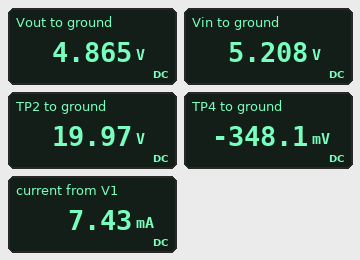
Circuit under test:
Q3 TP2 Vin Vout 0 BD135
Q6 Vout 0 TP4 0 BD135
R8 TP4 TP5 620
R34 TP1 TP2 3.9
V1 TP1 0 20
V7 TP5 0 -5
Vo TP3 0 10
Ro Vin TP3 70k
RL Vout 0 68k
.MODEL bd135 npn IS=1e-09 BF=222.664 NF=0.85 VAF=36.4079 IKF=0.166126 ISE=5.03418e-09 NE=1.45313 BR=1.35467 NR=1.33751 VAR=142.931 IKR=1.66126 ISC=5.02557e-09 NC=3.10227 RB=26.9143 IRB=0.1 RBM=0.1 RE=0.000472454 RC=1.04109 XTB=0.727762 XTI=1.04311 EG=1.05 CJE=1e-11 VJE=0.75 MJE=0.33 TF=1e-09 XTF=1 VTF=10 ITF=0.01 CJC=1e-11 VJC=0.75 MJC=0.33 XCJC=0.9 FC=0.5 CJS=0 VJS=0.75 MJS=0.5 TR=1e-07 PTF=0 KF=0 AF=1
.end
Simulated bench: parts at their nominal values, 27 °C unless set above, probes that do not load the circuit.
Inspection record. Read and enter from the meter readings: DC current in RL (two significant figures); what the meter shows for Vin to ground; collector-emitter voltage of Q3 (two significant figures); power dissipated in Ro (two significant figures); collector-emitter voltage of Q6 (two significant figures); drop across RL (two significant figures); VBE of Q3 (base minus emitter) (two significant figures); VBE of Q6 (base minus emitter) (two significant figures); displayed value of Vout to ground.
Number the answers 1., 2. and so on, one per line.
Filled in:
1. 72 µA
2. 5.208 V
3. 15 V
4. 330 µW
5. 5.2 V
6. 4.9 V
7. 340 mV
8. 350 mV
9. 4.865 V
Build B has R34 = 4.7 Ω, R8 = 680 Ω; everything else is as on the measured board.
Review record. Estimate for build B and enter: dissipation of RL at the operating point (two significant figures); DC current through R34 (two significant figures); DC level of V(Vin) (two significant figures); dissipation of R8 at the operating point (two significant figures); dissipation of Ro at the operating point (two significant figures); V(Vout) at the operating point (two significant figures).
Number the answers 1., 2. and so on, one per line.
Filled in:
1. 390 µW
2. 6.8 mA
3. 5.5 V
4. 32 mW
5. 290 µW
6. 5.2 V
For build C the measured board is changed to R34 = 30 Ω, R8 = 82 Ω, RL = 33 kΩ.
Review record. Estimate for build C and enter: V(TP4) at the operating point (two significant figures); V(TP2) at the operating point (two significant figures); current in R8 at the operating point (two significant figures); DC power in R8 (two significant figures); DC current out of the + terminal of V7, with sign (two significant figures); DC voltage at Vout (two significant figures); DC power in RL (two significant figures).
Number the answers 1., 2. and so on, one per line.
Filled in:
1. -920 mV
2. 19 V
3. 50 mA
4. 200 mW
5. -50 mA
6. -1.1 V
7. 36 µW
